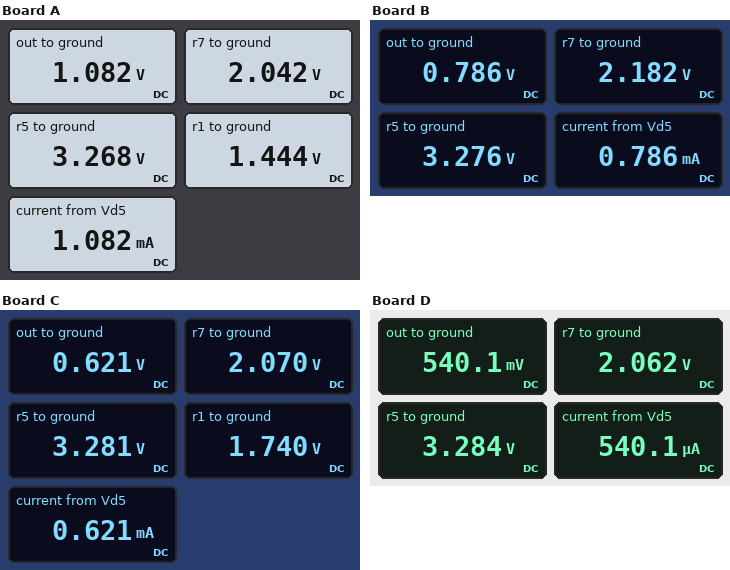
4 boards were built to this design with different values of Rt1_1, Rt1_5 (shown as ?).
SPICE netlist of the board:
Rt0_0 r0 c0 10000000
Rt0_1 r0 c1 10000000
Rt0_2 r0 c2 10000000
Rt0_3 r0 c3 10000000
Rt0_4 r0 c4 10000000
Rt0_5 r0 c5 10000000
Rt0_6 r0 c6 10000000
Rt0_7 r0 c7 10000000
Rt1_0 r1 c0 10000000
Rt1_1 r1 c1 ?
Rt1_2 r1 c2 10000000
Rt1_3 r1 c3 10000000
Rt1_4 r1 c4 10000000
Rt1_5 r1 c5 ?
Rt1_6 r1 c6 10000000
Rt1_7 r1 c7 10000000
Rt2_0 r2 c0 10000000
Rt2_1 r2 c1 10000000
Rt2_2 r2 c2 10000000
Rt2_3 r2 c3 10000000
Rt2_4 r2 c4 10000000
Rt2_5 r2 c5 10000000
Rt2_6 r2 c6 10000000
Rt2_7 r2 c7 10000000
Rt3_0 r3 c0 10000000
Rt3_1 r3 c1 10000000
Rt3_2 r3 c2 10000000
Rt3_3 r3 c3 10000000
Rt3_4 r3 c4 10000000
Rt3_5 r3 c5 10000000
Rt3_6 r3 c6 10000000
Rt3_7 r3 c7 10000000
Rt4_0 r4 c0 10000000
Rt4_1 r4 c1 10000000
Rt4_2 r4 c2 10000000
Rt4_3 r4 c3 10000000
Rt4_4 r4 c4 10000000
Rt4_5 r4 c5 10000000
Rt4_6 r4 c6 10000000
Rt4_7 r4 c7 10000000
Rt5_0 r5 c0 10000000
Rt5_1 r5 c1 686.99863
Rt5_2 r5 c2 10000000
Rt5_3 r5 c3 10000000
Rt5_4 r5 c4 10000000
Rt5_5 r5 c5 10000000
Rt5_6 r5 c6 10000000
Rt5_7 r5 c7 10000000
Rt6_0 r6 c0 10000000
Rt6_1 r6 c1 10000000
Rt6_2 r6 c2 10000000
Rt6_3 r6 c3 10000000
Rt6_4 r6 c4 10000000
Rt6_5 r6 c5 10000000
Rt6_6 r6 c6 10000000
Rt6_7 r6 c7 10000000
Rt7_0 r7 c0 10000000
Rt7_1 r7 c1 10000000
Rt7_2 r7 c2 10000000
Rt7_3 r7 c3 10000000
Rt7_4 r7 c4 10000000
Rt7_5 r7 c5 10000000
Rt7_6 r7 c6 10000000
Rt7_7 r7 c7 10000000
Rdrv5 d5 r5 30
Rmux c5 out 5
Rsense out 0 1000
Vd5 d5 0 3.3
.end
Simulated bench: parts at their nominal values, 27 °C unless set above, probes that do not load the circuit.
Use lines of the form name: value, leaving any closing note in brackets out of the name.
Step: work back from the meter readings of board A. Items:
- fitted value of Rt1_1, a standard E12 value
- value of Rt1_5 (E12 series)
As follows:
fitted value of Rt1_1, a standard E12 value: 1 kΩ
value of Rt1_5: 330 Ω
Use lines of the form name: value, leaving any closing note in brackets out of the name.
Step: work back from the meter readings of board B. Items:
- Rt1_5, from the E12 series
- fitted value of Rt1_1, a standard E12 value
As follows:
Rt1_5, from the E12 series: 1.8 kΩ
fitted value of Rt1_1, a standard E12 value: 680 Ω
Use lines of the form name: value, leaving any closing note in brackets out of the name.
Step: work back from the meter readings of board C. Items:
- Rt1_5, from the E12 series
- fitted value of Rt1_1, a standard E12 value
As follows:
Rt1_5, from the E12 series: 1.8 kΩ
fitted value of Rt1_1, a standard E12 value: 1.8 kΩ
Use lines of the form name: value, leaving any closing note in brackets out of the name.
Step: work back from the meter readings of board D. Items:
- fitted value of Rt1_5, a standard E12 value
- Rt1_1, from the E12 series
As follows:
fitted value of Rt1_5, a standard E12 value: 2.2 kΩ
Rt1_1, from the E12 series: 2.2 kΩ
